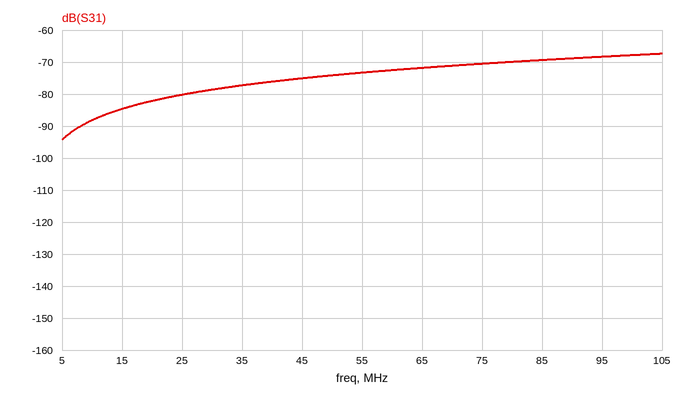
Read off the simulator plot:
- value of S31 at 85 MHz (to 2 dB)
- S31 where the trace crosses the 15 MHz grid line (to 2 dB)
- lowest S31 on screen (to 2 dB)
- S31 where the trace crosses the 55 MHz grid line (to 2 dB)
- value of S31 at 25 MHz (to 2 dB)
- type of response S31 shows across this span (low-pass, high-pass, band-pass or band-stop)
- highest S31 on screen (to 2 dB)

-70 dB
-84 dB
-94 dB
-74 dB
-80 dB
high-pass
-68 dB
